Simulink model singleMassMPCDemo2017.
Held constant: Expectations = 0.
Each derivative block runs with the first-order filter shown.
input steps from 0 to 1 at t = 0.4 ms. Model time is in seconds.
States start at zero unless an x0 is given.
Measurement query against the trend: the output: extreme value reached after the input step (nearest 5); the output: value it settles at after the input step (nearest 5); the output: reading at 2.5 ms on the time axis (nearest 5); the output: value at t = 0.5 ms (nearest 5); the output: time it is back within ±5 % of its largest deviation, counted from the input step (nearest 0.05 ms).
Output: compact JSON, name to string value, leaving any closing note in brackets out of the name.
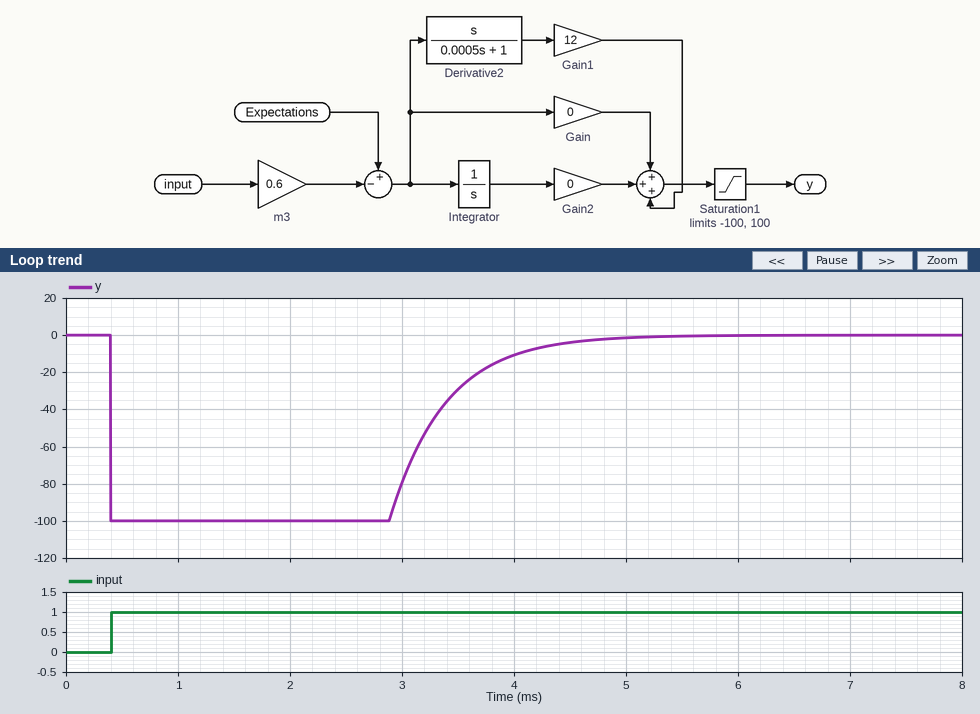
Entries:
{"the output: extreme value reached after the input step": "-100", "the output: value it settles at after the input step": "0", "the output: reading at 2.5 ms on the time axis": "-100", "the output: value at t = 0.5 ms": "-100", "the output: time it is back within ±5 % of its largest deviation, counted from the input step": "4.00 ms"}
